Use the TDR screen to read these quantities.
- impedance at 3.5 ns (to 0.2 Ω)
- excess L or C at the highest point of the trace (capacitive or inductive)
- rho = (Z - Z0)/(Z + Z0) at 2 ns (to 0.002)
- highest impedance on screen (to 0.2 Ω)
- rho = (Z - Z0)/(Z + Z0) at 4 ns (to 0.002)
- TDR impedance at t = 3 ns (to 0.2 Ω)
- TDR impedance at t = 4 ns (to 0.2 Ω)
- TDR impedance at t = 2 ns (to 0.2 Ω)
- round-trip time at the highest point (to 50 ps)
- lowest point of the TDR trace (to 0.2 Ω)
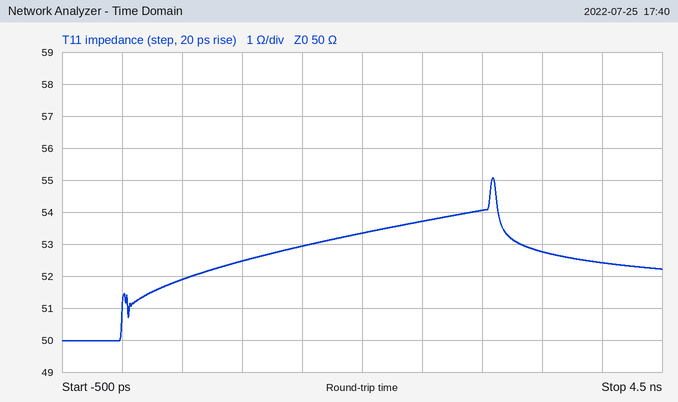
52.8 Ω
inductive
+0.032
55.0 Ω
+0.024
54.0 Ω
52.4 Ω
53.4 Ω
3.10 ns
50.0 Ω
